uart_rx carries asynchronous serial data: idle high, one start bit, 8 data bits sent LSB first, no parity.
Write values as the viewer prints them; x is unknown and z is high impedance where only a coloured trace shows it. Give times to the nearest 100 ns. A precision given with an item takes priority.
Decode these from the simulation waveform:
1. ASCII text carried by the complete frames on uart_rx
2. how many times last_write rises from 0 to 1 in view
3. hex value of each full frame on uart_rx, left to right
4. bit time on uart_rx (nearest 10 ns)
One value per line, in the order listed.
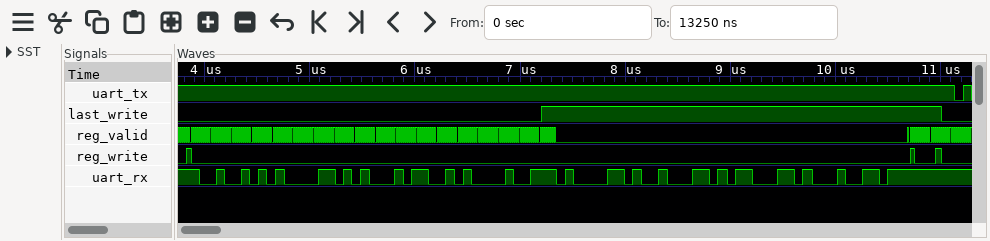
"RX4!abcd"
1
52, 58, 34, 21, 61, 62, 63, 64
80 ns
